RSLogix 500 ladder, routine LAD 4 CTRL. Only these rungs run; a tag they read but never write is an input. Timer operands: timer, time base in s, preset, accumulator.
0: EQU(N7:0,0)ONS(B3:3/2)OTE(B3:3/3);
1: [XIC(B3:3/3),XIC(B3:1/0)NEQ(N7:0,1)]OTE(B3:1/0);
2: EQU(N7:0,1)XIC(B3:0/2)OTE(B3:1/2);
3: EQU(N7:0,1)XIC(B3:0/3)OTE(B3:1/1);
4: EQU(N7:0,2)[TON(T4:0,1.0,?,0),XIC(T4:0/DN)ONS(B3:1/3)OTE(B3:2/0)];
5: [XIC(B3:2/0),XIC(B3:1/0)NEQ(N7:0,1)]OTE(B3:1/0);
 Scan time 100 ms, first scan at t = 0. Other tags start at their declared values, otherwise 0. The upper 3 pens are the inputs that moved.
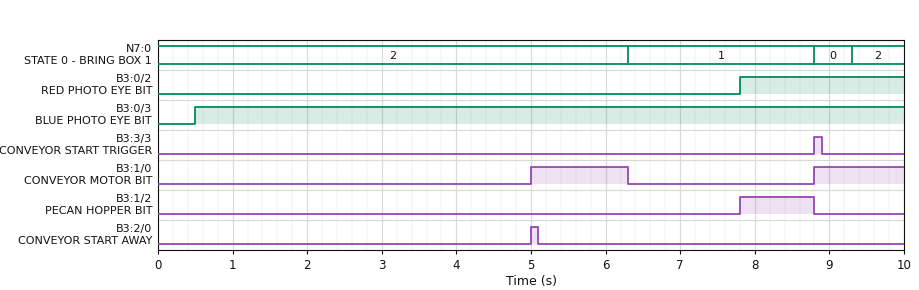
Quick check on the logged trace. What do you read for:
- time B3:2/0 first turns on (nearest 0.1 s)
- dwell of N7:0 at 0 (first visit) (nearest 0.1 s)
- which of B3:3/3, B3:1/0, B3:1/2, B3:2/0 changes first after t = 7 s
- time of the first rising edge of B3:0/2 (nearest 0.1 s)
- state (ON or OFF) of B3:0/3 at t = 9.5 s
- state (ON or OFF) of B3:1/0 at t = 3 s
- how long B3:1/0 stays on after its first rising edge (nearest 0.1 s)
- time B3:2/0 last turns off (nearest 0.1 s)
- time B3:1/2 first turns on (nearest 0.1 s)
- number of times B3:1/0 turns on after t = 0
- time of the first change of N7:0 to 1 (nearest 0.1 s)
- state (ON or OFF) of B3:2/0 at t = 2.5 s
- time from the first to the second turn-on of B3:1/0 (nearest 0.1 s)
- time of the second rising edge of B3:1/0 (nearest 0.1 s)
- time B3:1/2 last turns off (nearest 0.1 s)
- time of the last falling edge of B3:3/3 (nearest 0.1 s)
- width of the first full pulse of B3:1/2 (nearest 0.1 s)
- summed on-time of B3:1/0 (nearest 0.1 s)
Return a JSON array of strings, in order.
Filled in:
["5.0 s", "0.5 s", "B3:1/2", "7.8 s", "ON", "OFF", "1.3 s", "5.1 s", "7.8 s", "2", "6.3 s", "OFF", "3.8 s", "8.8 s", "8.8 s", "8.9 s", "1.0 s", "2.5 s"]
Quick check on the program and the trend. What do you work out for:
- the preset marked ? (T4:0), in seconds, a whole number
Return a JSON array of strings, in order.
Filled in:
["5 s"]
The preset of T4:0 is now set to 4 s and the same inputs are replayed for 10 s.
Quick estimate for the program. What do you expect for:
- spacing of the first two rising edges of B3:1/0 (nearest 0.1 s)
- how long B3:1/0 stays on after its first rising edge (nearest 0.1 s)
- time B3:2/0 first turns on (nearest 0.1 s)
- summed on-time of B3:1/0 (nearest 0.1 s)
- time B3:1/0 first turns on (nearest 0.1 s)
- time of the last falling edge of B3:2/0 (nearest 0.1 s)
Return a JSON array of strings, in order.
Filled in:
["4.8 s", "2.3 s", "4.0 s", "3.5 s", "4.0 s", "4.1 s"]
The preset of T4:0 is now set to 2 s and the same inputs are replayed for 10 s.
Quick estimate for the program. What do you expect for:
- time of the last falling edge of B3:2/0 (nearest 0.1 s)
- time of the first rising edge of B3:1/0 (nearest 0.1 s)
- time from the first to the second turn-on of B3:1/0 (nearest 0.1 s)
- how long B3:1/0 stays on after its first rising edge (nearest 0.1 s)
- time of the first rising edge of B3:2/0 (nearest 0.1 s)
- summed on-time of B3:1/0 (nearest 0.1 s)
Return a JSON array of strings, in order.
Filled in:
["2.1 s", "2.0 s", "6.8 s", "4.3 s", "2.0 s", "5.5 s"]
